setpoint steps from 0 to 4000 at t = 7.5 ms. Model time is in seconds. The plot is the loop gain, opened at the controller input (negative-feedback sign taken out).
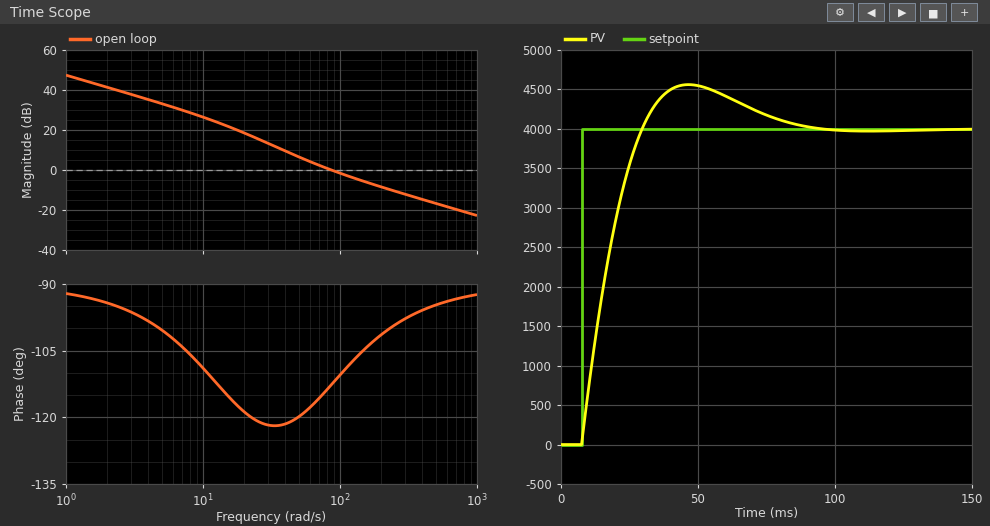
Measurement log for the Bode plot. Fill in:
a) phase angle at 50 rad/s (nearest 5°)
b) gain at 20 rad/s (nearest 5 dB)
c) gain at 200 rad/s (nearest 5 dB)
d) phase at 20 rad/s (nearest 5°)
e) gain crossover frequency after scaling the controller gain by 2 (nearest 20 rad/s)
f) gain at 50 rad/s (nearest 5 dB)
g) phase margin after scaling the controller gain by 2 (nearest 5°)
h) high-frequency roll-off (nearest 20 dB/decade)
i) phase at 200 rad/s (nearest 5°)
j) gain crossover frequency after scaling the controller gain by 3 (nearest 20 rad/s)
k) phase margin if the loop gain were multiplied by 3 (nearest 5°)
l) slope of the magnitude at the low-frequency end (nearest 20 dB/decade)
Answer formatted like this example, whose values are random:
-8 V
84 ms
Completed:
-120°
20 dB
-10 dB
-120°
160 rad/s
5 dB
75°
-20 dB/decade
-100°
220 rad/s
80°
-20 dB/decade
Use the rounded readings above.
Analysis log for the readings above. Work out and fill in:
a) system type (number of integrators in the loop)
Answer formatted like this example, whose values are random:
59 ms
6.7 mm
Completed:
1
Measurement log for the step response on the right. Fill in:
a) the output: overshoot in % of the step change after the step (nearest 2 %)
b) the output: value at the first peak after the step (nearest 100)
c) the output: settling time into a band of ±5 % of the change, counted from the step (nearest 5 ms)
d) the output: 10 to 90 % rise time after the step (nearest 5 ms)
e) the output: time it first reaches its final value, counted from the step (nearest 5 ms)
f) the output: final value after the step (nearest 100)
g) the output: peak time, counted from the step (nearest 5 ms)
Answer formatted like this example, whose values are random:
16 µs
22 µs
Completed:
14 %
4600
65 ms
15 ms
20 ms
4000
40 ms
